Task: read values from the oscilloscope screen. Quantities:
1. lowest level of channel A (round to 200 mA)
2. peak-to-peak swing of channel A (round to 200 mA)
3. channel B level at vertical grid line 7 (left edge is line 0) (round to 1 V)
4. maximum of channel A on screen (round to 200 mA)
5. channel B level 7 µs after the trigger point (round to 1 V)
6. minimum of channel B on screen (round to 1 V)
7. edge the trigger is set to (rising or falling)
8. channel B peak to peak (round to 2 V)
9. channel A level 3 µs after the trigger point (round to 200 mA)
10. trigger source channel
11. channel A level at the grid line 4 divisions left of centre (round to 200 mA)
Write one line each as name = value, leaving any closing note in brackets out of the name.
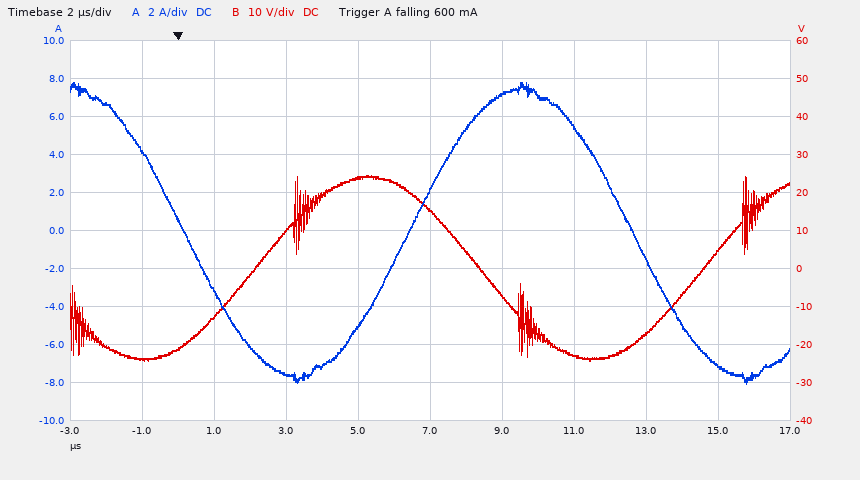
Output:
lowest level of channel A = -8.0 A
peak-to-peak swing of channel A = 15.8 A
channel B level at vertical grid line 7 (left edge is line 0) = -23 V
maximum of channel A on screen = 7.8 A
channel B level 7 µs after the trigger point = 15 V
minimum of channel B on screen = -24 V
edge the trigger is set to = falling
channel B peak to peak = 48 V
channel A level 3 µs after the trigger point = -7.6 A
trigger source channel = channel A
channel A level at the grid line 4 divisions left of centre = 4.2 A
